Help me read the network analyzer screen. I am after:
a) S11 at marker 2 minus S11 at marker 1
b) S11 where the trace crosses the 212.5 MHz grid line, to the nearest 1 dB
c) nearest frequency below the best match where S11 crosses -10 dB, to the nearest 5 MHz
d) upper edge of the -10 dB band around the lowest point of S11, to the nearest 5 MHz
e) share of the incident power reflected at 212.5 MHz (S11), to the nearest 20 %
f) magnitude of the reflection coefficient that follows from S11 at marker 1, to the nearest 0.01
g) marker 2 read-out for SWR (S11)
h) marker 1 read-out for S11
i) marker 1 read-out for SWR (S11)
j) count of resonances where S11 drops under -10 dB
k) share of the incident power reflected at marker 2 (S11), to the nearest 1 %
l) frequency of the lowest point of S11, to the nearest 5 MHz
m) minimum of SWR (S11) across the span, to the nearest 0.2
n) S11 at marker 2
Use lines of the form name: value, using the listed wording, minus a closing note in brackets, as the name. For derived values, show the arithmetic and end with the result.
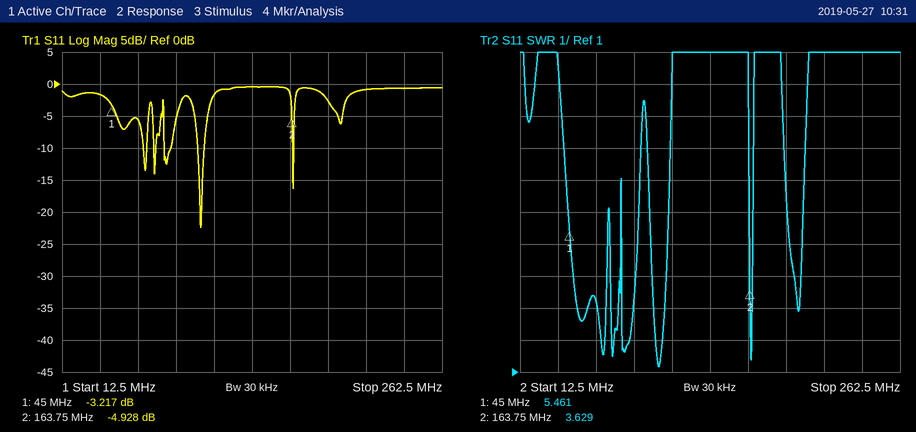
S11 at marker 2 minus S11 at marker 1: -4.928 − (-3.217) = -1.711 dB
S11 where the trace crosses the 212.5 MHz grid line, to the nearest 1 dB: -1 dB
nearest frequency below the best match where S11 crosses -10 dB, to the nearest 5 MHz: 100 MHz
upper edge of the -10 dB band around the lowest point of S11, to the nearest 5 MHz: 105 MHz
share of the incident power reflected at 212.5 MHz (S11), to the nearest 20 %: 10^(-1/10) ≈ 79.4 %, so 80 % to the nearest 20 %
magnitude of the reflection coefficient that follows from S11 at marker 1, to the nearest 0.01: 10^(-3.217/20) ≈ 0.69
marker 2 read-out for SWR: 3.629
marker 1 read-out for S11: -3.217 dB
marker 1 read-out for SWR: 5.461
count of resonances where S11 drops under -10 dB: 5
share of the incident power reflected at marker 2 (S11), to the nearest 1 %: 10^(-4.928/10) ≈ 32 %
frequency of the lowest point of S11, to the nearest 5 MHz: 105 MHz
minimum of SWR (S11) across the span, to the nearest 0.2: 1.2
S11 at marker 2: -4.928 dB
